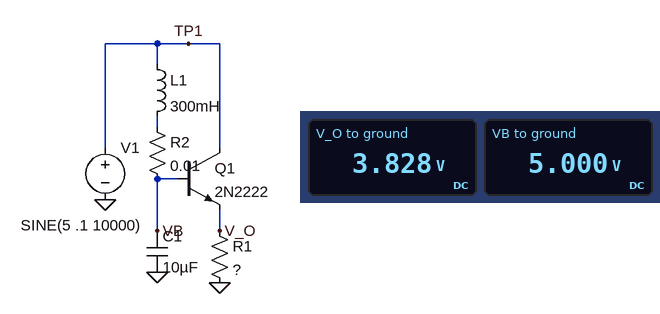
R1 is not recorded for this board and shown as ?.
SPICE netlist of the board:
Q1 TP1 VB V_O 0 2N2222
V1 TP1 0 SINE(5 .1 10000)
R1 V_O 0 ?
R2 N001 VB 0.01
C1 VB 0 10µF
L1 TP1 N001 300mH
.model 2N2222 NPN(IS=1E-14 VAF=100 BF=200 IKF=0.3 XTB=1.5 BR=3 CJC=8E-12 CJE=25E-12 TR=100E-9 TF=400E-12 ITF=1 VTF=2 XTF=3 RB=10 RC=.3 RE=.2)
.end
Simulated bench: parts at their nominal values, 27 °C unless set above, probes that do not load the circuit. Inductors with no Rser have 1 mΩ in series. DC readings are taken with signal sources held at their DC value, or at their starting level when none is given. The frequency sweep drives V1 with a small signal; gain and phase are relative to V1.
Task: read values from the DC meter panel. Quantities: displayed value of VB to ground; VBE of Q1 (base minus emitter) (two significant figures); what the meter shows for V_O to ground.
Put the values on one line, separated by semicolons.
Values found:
5.000 V; 1.2 V; 3.828 V
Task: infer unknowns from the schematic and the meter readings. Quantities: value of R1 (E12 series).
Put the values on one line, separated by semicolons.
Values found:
4.7 Ω
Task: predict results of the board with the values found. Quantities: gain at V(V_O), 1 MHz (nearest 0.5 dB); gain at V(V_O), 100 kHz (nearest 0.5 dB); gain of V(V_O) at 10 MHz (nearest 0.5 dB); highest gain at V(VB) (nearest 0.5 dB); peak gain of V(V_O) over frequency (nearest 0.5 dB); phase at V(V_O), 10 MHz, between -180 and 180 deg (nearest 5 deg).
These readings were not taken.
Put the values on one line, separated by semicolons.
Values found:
-39.0 dB; -51.0 dB; -20.0 dB; 1.0 dB; 0 dB; 65 deg
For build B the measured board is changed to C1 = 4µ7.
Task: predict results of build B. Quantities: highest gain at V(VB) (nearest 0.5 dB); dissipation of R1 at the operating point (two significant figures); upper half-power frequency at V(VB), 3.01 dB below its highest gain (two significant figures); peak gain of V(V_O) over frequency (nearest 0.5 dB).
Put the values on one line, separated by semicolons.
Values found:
0 dB; 3.1 W; 120 Hz; -1.0 dB
